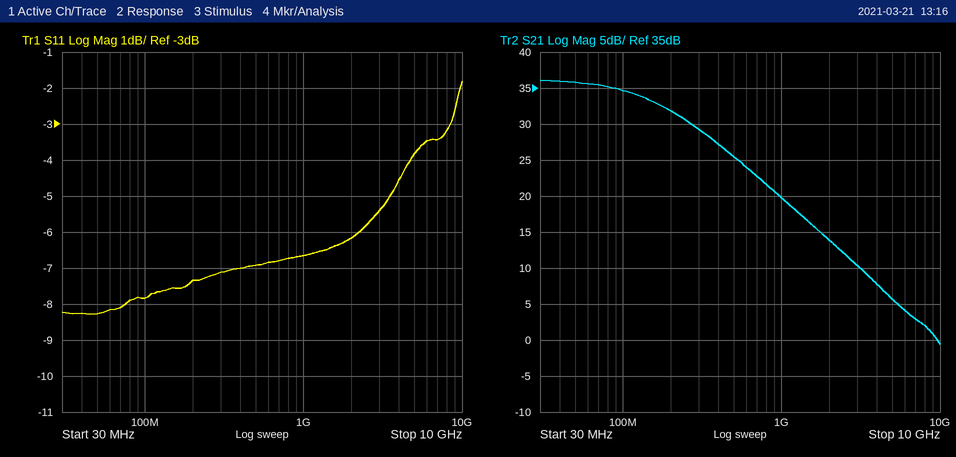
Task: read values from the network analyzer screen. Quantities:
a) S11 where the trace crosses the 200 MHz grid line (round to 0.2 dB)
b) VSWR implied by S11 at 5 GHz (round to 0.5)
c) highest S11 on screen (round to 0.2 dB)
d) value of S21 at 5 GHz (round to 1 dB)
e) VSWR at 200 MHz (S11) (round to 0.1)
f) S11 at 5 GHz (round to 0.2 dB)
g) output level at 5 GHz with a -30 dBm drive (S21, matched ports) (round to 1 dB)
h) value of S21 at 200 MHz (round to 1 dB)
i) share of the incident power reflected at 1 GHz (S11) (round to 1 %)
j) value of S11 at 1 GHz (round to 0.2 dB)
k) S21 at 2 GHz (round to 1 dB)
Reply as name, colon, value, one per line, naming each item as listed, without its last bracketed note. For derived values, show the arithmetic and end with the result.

S11 where the trace crosses the 200 MHz grid line: -7.4 dB
VSWR implied by S11 at 5 GHz: |Γ| = 10^(-3.8/20) = 0.6457; VSWR = (1 + 0.6457)/(1 − 0.6457) ≈ 4.64, so 4.5 to the nearest 0.5
highest S11 on screen: -1.8 dB
value of S21 at 5 GHz: 6 dB
VSWR at 200 MHz (S11): |Γ| = 10^(-7.4/20) = 0.4266; VSWR = (1 + 0.4266)/(1 − 0.4266) ≈ 2.5
S11 at 5 GHz: -3.8 dB
output level at 5 GHz with a -30 dBm drive (S21, matched ports): -30 dBm + (6 dB) = -24 dBm
value of S21 at 200 MHz: 32 dB
share of the incident power reflected at 1 GHz (S11): 10^(-6.6/10) ≈ 22 %
value of S11 at 1 GHz: -6.6 dB
S21 at 2 GHz: 14 dB
